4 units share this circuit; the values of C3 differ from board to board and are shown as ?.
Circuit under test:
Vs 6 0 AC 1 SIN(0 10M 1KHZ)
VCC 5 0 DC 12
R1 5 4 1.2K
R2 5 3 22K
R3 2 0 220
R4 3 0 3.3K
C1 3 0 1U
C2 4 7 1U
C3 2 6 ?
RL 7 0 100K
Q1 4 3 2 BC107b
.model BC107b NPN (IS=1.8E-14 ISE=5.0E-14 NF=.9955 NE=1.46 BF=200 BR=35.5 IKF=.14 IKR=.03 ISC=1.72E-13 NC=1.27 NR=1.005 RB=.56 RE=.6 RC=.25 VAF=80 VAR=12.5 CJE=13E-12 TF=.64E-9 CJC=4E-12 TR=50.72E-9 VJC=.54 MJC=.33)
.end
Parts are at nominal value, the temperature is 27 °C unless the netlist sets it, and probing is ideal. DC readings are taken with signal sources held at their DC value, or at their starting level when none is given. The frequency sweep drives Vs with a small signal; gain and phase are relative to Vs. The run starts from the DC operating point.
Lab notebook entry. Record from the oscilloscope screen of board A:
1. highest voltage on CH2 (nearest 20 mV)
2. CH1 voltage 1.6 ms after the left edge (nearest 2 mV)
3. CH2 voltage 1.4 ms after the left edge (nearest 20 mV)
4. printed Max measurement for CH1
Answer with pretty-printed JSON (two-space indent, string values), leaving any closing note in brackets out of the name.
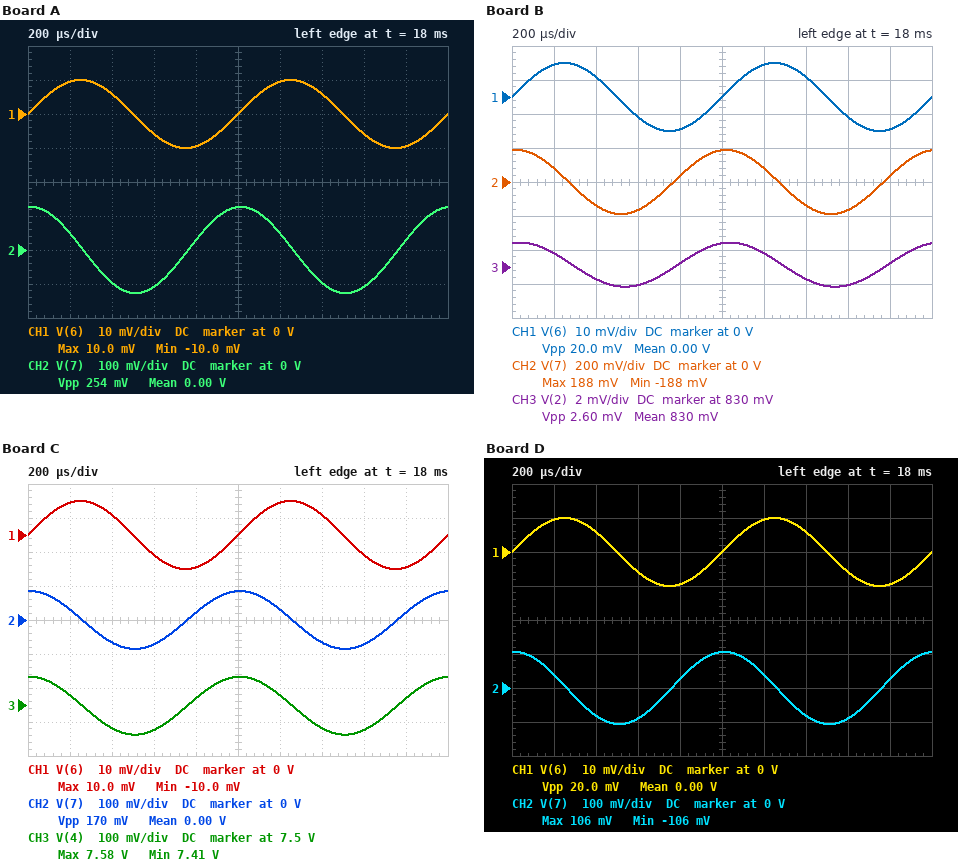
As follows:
{
  "highest voltage on CH2": "120 mV",
  "CH1 voltage 1.6 ms after the left edge": "-6 mV",
  "CH2 voltage 1.4 ms after the left edge": "-100 mV",
  "printed Max measurement for CH1": "10.0 mV"
}
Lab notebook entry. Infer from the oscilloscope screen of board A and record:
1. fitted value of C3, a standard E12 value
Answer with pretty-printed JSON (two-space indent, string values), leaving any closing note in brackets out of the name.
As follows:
{
  "fitted value of C3, a standard E12 value": "1.8 µF"
}
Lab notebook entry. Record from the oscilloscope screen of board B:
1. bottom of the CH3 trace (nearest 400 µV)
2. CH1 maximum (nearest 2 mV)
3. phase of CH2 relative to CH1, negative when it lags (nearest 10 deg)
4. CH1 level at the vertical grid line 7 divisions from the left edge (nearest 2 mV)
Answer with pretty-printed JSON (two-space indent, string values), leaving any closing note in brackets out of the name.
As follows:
{
  "bottom of the CH3 trace": "828.8 mV",
  "CH1 maximum": "10 mV",
  "phase of CH2 relative to CH1, negative when it lags": "80 deg",
  "CH1 level at the vertical grid line 7 divisions from the left edge": "6 mV"
}
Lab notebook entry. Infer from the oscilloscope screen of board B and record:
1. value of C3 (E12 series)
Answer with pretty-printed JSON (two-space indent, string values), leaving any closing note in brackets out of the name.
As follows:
{
  "value of C3": "2.7 µF"
}
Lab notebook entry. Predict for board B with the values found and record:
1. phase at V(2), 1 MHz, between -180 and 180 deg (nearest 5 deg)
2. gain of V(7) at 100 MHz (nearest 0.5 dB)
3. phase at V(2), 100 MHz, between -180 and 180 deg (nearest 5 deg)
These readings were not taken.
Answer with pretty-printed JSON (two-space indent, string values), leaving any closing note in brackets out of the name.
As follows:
{
  "phase at V(2), 1 MHz, between -180 and 180 deg": "0 deg",
  "gain of V(7) at 100 MHz": "39.0 dB",
  "phase at V(2), 100 MHz, between -180 and 180 deg": "0 deg"
}
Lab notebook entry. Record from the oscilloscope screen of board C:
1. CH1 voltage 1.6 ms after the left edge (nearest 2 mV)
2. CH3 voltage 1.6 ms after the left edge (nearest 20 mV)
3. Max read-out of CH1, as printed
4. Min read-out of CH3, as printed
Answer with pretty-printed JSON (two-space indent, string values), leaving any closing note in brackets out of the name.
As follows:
{
  "CH1 voltage 1.6 ms after the left edge": "-6 mV",
  "CH3 voltage 1.6 ms after the left edge": "7.42 V",
  "Max read-out of CH1, as printed": "10.0 mV",
  "Min read-out of CH3, as printed": "7.41 V"
}
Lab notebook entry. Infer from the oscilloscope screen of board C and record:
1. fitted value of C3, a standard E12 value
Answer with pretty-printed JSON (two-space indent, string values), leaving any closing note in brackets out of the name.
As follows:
{
  "fitted value of C3, a standard E12 value": "1.2 µF"
}
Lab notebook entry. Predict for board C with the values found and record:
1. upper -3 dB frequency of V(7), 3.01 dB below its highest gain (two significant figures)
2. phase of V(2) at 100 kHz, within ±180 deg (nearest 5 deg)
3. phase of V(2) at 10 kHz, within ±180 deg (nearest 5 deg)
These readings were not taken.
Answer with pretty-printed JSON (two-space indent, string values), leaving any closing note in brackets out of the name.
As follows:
{
  "upper -3 dB frequency of V(7), 3.01 dB below its highest gain": "74 MHz",
  "phase of V(2) at 100 kHz, within ±180 deg": "10 deg",
  "phase of V(2) at 10 kHz, within ±180 deg": "60 deg"
}
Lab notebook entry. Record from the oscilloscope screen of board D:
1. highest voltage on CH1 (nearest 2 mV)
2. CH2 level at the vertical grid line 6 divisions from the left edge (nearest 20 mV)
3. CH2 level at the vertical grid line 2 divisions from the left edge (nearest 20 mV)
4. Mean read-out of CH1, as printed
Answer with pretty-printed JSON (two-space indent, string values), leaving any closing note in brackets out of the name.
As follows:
{
  "highest voltage on CH1": "10 mV",
  "CH2 level at the vertical grid line 6 divisions from the left edge": "40 mV",
  "CH2 level at the vertical grid line 2 divisions from the left edge": "-80 mV",
  "Mean read-out of CH1, as printed": "0.00 V"
}
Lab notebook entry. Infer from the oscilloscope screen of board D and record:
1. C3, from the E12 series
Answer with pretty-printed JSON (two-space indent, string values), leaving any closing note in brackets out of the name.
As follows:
{
  "C3, from the E12 series": "1.5 µF"
}
